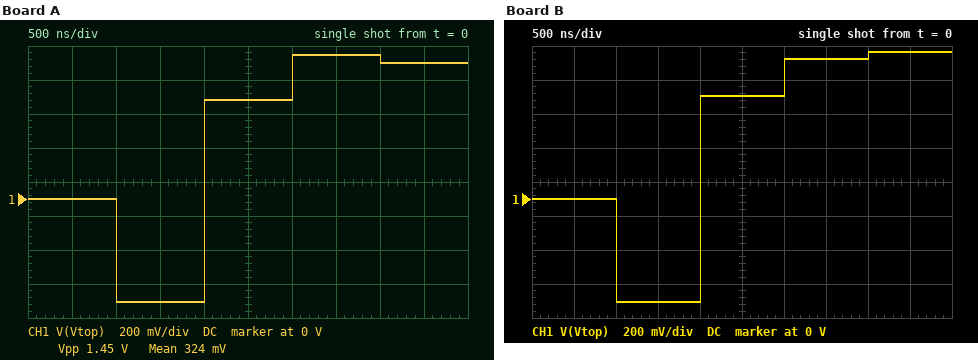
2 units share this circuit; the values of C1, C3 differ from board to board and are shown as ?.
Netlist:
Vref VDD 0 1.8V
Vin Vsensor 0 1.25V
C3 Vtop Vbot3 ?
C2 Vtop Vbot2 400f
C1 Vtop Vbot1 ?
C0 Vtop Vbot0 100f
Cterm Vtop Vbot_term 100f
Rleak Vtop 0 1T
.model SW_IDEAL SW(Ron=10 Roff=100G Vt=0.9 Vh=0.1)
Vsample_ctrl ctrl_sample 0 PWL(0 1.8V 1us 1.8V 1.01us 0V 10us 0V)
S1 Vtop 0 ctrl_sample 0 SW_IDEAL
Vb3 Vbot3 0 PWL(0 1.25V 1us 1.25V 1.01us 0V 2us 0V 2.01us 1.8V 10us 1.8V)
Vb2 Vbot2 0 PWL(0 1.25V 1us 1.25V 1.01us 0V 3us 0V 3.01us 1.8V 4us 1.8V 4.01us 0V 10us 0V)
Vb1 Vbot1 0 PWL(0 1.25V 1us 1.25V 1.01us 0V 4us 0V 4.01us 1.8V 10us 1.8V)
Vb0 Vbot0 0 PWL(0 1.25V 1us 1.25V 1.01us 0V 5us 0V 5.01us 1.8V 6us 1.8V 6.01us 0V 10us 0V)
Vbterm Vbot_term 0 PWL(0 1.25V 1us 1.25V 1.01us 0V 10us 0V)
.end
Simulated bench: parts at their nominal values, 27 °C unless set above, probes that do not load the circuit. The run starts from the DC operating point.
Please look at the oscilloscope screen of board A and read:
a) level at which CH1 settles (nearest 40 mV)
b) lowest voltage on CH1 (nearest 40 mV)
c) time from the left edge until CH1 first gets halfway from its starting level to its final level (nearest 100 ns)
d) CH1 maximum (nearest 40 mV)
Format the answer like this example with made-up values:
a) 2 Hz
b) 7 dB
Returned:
a) 800 mV
b) -600 mV
c) 2.0 µs
d) 840 mV
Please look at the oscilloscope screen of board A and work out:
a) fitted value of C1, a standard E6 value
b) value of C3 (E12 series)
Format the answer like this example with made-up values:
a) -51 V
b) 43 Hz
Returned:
a) 330 fF
b) 1.8 pF
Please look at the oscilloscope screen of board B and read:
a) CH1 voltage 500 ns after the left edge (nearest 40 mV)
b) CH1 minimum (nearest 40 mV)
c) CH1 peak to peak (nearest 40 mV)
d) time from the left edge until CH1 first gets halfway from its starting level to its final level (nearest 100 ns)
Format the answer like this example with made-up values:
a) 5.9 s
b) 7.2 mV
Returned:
a) 0 V
b) -600 mV
c) 1.48 V
d) 2.0 µs
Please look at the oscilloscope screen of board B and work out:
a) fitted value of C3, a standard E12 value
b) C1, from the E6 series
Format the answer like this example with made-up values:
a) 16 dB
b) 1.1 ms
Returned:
a) 2.2 pF
b) 470 fF
